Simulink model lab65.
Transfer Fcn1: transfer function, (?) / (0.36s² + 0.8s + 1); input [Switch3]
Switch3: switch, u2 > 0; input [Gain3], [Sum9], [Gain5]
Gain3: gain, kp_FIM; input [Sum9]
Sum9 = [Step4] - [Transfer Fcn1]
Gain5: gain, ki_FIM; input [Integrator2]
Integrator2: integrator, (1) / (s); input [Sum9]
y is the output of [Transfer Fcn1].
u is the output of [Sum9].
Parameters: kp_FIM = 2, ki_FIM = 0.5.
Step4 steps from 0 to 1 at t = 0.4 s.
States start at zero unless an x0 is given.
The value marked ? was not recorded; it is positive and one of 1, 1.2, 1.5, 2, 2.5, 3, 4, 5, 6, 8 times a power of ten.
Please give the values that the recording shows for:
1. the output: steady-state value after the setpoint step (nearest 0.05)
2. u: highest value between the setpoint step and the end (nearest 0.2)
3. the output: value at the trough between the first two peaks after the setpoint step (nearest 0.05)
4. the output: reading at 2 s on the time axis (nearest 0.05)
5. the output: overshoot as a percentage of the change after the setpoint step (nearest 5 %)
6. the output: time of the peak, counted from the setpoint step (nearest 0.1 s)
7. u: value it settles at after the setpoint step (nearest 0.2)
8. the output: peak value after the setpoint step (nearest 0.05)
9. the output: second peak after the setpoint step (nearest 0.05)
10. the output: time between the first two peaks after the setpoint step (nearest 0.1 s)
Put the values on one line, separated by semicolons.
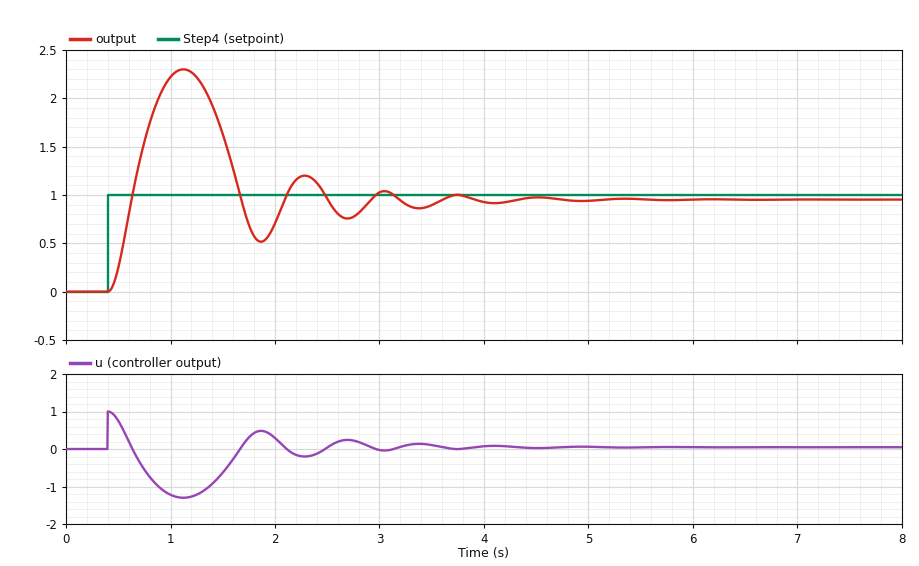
0.95; 1.0; 0.50; 0.70; 140 %; 0.7 s; 0.0; 2.30; 1.20; 1.2 s
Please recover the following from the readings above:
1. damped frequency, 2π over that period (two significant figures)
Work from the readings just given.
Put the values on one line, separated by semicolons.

5.2 rad/s
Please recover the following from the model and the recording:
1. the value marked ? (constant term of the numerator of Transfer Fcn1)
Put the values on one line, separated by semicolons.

10
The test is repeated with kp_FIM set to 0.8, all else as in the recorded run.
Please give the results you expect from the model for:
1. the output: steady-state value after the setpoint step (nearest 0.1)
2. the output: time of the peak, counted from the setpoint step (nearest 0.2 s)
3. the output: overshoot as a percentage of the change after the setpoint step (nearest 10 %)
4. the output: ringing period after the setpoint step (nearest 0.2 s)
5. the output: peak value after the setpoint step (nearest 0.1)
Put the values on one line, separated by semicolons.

0.9; 1.0 s; 90 %; 1.6 s; 1.7
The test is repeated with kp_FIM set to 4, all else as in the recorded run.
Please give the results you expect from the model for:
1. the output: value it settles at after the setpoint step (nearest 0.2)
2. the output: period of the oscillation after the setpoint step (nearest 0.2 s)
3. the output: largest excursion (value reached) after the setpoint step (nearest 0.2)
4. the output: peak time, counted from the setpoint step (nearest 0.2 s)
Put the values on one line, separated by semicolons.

1.0; 1.0 s; 3.0; 0.6 s
